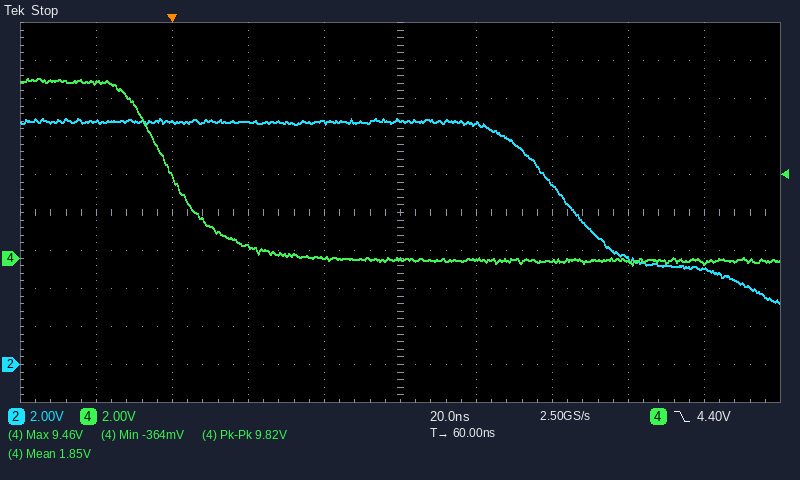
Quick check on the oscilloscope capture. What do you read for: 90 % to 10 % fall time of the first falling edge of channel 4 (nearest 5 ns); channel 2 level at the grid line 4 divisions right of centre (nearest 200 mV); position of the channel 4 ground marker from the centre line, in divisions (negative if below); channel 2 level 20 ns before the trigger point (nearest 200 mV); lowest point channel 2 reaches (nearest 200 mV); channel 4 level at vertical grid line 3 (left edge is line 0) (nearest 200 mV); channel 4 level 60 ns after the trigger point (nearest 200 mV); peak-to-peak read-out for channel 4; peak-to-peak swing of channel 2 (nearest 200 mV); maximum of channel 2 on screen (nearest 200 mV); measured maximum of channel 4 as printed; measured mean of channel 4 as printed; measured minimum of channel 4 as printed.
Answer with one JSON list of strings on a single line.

["30 ns", "5.0 V", "-1.2 div", "12.8 V", "3.2 V", "600 mV", "0.0 V", "9.82 V", "9.8 V", "13.0 V", "9.46 V", "1.85 V", "-364 mV"]
